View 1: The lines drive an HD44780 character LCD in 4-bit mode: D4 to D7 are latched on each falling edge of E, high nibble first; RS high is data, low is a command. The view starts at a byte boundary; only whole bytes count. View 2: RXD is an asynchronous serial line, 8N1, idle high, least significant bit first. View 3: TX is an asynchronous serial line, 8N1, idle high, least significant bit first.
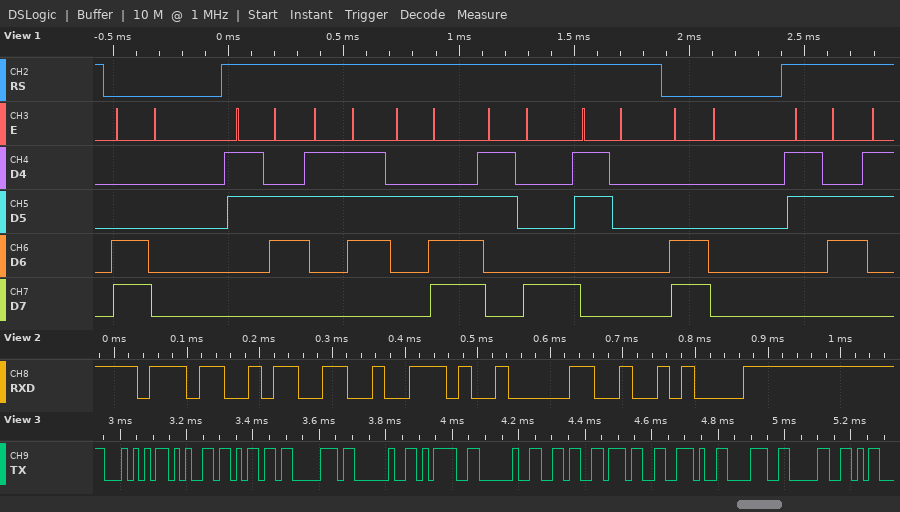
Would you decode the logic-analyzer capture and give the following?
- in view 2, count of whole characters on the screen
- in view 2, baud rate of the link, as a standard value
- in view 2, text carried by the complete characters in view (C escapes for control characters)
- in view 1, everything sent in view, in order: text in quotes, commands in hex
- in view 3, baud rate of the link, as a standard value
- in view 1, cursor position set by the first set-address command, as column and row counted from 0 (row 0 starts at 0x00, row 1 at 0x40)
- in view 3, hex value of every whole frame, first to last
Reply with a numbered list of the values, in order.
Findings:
1. 5
2. 57600 baud
3. "73.0\n"
4. 0xC0 "67.80" 0xC0 "6"
5. 57600 baud
6. column 0, row 1
7. 54 65 6D 70 20 3D 20 36 37 2E 38 30
